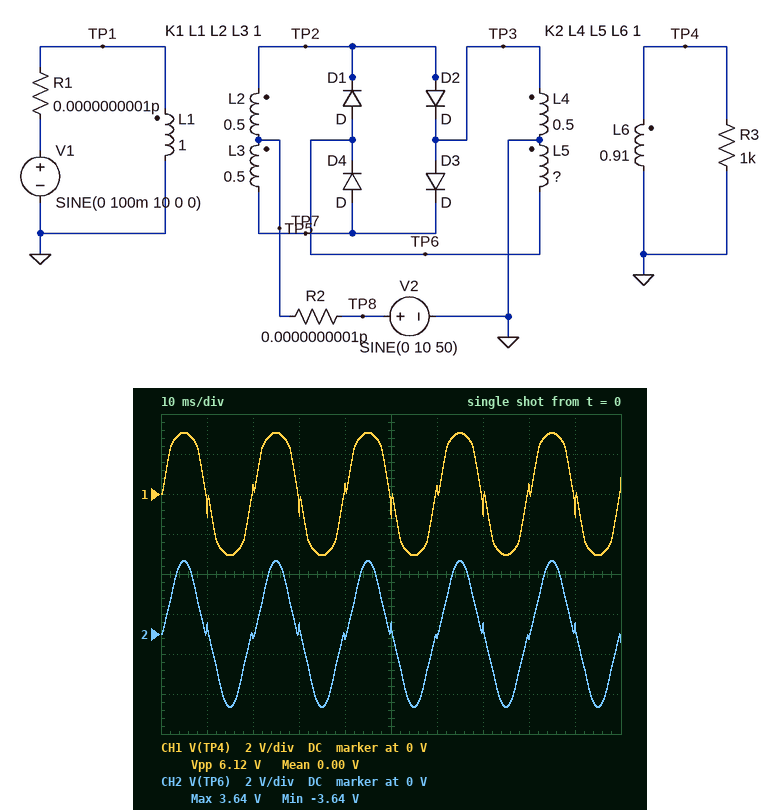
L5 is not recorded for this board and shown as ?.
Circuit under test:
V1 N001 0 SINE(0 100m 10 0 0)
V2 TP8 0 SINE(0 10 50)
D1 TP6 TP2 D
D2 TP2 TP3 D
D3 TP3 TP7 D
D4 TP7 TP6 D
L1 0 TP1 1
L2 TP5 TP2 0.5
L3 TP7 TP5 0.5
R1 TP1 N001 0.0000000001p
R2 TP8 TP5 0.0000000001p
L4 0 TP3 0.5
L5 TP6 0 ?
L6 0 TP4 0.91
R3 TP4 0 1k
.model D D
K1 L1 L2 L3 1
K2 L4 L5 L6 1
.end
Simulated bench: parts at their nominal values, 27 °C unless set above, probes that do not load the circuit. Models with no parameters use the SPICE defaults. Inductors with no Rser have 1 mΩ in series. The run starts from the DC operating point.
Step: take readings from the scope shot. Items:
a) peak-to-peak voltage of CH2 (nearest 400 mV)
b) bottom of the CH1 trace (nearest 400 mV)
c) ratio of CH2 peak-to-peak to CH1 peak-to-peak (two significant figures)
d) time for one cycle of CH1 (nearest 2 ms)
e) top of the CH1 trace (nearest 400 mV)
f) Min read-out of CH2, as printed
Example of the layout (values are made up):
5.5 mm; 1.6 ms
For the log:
7.2 V; -3.2 V; 1.2; 20 ms; 3.2 V; -3.64 V
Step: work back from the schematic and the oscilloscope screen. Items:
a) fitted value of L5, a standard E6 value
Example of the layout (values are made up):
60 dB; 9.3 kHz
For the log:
220 mH
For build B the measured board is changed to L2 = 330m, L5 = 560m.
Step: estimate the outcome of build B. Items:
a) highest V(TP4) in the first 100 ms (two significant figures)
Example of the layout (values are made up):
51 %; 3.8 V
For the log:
1.0 V
